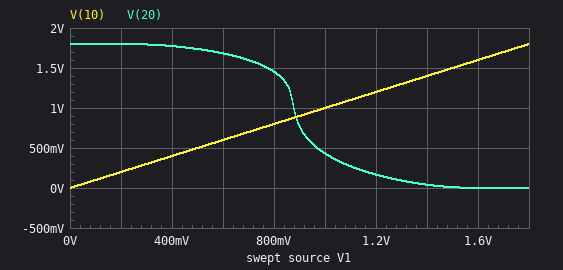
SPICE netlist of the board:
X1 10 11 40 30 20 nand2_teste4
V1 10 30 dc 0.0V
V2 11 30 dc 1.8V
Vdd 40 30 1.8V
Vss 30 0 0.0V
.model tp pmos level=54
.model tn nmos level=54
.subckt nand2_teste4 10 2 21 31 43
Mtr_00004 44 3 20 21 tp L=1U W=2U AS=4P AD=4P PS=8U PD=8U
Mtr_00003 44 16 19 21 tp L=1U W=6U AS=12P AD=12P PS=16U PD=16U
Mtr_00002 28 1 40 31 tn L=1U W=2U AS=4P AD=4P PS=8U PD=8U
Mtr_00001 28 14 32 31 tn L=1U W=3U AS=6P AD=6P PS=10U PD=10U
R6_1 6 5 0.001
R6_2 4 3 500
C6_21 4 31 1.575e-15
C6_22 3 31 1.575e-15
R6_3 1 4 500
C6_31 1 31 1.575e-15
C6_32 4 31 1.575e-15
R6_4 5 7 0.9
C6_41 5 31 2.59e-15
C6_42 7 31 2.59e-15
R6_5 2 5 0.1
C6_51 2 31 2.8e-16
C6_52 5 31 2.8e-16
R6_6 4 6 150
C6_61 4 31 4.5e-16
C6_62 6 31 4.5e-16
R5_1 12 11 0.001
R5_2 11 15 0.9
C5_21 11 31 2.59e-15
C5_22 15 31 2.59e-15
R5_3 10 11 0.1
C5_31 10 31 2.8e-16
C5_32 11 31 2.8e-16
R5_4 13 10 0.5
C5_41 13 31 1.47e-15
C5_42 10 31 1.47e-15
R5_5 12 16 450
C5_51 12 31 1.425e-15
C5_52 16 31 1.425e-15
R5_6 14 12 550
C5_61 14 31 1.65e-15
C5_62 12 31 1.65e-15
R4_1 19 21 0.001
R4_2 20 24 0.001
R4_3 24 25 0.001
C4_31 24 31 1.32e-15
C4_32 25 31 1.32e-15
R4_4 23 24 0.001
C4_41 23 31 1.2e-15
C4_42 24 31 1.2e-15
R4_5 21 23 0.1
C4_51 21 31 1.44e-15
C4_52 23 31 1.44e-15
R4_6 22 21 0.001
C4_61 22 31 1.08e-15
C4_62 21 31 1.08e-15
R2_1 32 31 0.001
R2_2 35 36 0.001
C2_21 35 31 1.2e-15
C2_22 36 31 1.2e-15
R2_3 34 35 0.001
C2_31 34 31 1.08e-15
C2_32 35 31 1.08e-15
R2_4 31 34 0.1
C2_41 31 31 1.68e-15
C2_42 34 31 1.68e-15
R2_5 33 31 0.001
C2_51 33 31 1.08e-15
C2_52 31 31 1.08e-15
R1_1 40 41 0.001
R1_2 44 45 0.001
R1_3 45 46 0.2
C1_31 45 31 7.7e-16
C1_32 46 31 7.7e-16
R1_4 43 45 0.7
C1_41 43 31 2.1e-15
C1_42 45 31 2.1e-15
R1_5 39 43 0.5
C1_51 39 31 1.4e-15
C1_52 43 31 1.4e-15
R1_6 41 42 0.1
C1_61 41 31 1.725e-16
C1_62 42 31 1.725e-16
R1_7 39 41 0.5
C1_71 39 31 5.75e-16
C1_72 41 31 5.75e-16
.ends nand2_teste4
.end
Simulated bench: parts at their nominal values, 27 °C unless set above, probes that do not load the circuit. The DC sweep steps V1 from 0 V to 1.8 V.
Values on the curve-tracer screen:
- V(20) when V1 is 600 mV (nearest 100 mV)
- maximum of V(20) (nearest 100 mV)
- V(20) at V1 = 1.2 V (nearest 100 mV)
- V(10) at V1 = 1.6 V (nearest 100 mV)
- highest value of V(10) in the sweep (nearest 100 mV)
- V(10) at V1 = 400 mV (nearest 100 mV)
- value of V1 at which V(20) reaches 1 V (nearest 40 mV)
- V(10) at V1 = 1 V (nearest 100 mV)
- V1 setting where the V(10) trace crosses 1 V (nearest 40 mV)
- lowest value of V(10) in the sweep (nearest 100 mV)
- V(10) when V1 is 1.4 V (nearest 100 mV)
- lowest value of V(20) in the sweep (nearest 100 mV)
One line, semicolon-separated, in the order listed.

1.7 V; 1.8 V; 200 mV; 1.6 V; 1.8 V; 400 mV; 880 mV; 1.0 V; 1.00 V; 0 V; 1.4 V; 0 V
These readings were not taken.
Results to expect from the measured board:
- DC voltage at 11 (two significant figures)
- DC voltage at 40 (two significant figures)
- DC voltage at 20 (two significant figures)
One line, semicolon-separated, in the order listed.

1.8 V; 1.8 V; 1.8 V
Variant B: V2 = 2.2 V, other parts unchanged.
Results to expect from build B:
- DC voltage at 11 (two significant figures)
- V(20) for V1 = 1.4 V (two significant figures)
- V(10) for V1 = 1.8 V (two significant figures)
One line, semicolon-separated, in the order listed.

2.2 V; 38 mV; 1.8 V
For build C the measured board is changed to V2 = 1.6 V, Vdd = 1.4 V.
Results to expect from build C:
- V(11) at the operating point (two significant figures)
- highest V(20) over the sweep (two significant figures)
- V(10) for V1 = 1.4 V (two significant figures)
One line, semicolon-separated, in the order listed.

1.6 V; 1.4 V; 1.4 V
